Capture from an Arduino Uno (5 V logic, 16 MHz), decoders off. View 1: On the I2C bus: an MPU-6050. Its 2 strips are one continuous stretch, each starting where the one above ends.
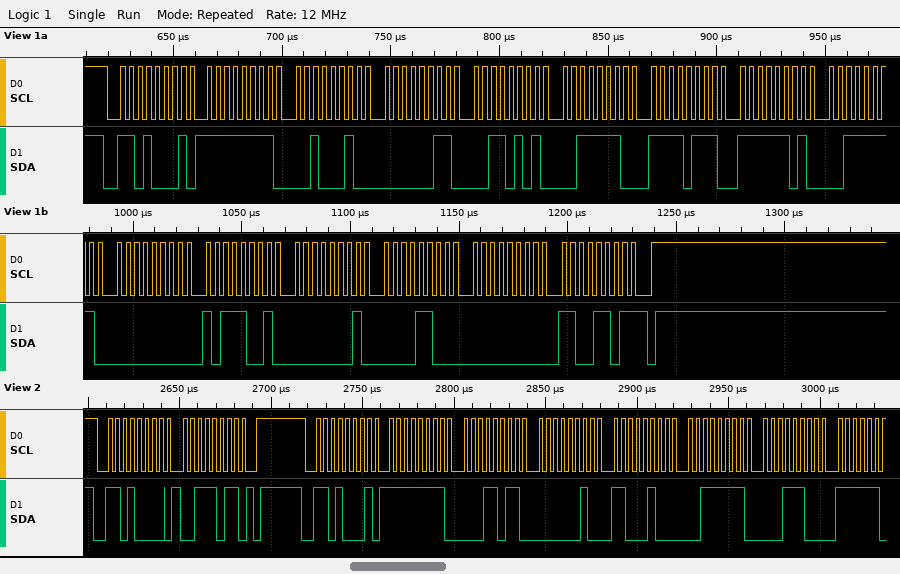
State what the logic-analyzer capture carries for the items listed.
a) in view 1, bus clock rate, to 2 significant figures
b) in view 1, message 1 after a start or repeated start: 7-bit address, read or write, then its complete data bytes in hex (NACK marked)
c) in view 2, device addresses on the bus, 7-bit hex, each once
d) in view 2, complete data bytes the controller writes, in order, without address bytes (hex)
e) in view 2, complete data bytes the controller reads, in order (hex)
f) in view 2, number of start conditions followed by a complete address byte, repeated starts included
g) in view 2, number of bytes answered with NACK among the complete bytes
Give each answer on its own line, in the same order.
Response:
250 kHz
0x68 read: FF 22 03 35 3E F7 FD 3F 00 B9 01 0C 00 CD NACK
0x68
3B
FF 1B 02 C4 3F 1C
2
0
